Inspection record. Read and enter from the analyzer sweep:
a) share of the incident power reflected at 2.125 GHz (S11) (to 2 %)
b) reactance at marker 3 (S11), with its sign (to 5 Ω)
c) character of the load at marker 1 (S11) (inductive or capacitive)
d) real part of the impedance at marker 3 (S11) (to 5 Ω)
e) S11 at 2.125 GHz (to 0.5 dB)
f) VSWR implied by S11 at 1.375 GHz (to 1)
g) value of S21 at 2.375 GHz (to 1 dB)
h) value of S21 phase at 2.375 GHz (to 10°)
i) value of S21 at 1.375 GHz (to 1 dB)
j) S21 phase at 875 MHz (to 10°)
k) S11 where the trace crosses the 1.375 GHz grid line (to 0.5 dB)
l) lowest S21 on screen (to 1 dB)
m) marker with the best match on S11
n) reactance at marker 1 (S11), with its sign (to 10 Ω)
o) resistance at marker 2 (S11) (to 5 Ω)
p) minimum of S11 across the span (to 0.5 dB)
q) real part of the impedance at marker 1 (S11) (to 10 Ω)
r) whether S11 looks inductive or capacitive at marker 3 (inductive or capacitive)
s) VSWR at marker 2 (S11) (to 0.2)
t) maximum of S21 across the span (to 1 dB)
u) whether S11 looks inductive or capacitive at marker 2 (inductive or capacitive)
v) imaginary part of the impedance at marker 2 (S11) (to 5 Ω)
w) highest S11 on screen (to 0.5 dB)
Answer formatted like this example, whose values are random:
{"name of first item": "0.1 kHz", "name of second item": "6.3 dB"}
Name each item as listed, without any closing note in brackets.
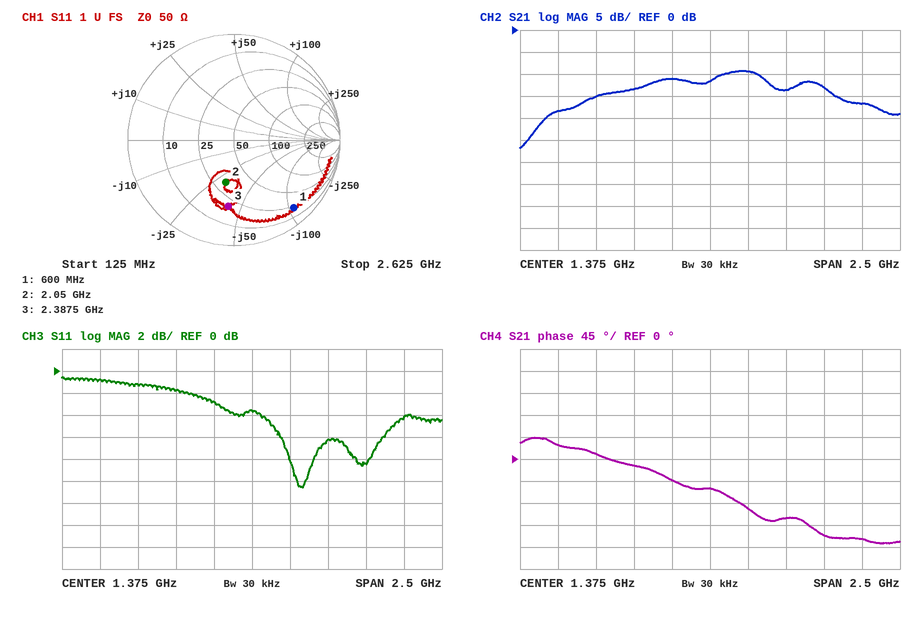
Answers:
{"share of the incident power reflected at 2.125 GHz (S11)": "14 %", "reactance at marker 3 (S11), with its sign": "-40 Ω", "character of the load at marker 1 (S11)": "capacitive", "real part of the impedance at marker 3 (S11)": "20 Ω", "S11 at 2.125 GHz": "-8.5 dB", "VSWR implied by S11 at 1.375 GHz": "5", "value of S21 at 2.375 GHz": "-17 dB", "value of S21 phase at 2.375 GHz": "-160°", "value of S21 at 1.375 GHz": "-12 dB", "S21 phase at 875 MHz": "-10°", "S11 where the trace crosses the 1.375 GHz grid line": "-3.5 dB", "lowest S21 on screen": "-27 dB", "marker with the best match on S11": "marker 2", "reactance at marker 1 (S11), with its sign": "-110 Ω", "resistance at marker 2 (S11)": "30 Ω", "minimum of S11 across the span": "-10.5 dB", "real part of the impedance at marker 1 (S11)": "20 Ω", "whether S11 looks inductive or capacitive at marker 3": "capacitive", "VSWR at marker 2 (S11)": "2.4", "maximum of S21 across the span": "-9 dB", "whether S11 looks inductive or capacitive at marker 2": "capacitive", "imaginary part of the impedance at marker 2 (S11)": "-30 Ω", "highest S11 on screen": "-0.5 dB"}
